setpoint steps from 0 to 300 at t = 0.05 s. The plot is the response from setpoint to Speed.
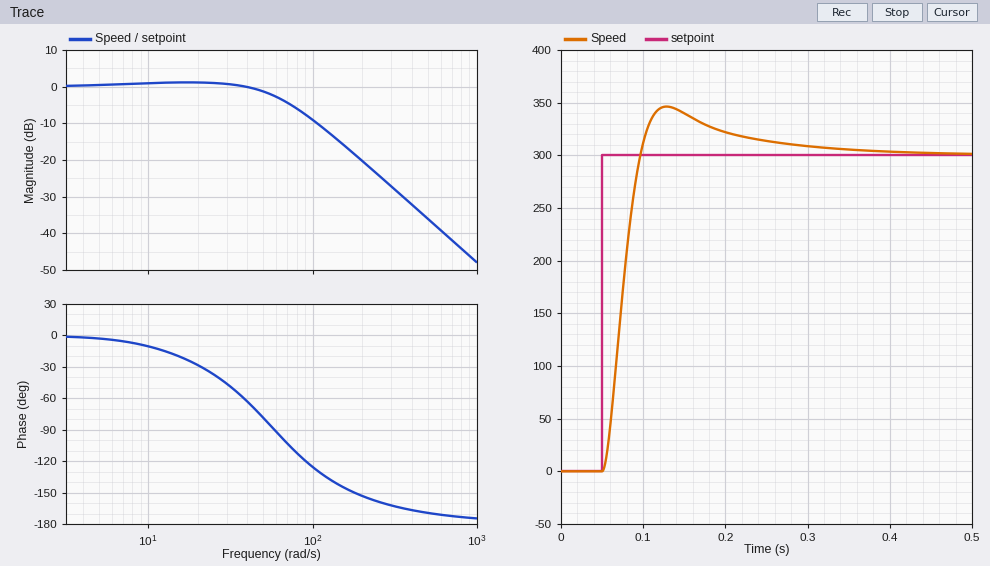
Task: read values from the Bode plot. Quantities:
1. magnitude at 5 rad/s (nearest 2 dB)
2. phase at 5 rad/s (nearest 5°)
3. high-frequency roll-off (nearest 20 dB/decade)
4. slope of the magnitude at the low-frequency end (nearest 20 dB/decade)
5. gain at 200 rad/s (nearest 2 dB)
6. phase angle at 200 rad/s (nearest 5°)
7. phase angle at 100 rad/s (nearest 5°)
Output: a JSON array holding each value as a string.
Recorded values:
["0 dB", "-5°", "-40 dB/decade", "0 dB/decade", "-20 dB", "-155°", "-125°"]
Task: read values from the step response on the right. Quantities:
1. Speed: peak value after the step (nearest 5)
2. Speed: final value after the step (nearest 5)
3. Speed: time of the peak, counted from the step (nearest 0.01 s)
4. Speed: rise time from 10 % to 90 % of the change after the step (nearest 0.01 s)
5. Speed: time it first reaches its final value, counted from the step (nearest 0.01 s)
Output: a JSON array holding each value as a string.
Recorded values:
["345", "300", "0.08 s", "0.03 s", "0.05 s"]
